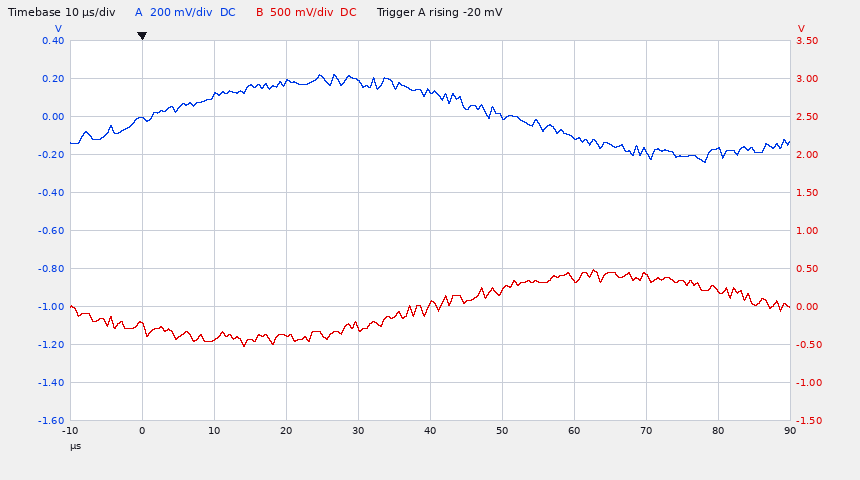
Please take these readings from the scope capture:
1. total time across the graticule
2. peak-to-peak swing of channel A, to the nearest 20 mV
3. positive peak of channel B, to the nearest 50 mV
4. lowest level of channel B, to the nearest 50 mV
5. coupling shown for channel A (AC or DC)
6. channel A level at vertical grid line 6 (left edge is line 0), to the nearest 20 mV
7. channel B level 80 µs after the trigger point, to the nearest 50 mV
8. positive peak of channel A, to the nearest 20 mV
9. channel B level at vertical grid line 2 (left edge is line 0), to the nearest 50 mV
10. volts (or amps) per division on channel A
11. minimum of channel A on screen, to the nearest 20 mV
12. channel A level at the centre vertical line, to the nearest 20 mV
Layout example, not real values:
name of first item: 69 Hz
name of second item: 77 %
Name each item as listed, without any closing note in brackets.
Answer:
total time across the graticule: 100 µs
peak-to-peak swing of channel A, to the nearest 20 mV: 460 mV
positive peak of channel B, to the nearest 50 mV: 500 mV
lowest level of channel B, to the nearest 50 mV: -550 mV
coupling shown for channel A: DC
channel A level at vertical grid line 6 (left edge is line 0), to the nearest 20 mV: 0 mV
channel B level 80 µs after the trigger point, to the nearest 50 mV: 200 mV
positive peak of channel A, to the nearest 20 mV: 220 mV
channel B level at vertical grid line 2 (left edge is line 0), to the nearest 50 mV: -450 mV
volts (or amps) per division on channel A: 200 mV
minimum of channel A on screen, to the nearest 20 mV: -240 mV
channel A level at the centre vertical line, to the nearest 20 mV: 140 mV
